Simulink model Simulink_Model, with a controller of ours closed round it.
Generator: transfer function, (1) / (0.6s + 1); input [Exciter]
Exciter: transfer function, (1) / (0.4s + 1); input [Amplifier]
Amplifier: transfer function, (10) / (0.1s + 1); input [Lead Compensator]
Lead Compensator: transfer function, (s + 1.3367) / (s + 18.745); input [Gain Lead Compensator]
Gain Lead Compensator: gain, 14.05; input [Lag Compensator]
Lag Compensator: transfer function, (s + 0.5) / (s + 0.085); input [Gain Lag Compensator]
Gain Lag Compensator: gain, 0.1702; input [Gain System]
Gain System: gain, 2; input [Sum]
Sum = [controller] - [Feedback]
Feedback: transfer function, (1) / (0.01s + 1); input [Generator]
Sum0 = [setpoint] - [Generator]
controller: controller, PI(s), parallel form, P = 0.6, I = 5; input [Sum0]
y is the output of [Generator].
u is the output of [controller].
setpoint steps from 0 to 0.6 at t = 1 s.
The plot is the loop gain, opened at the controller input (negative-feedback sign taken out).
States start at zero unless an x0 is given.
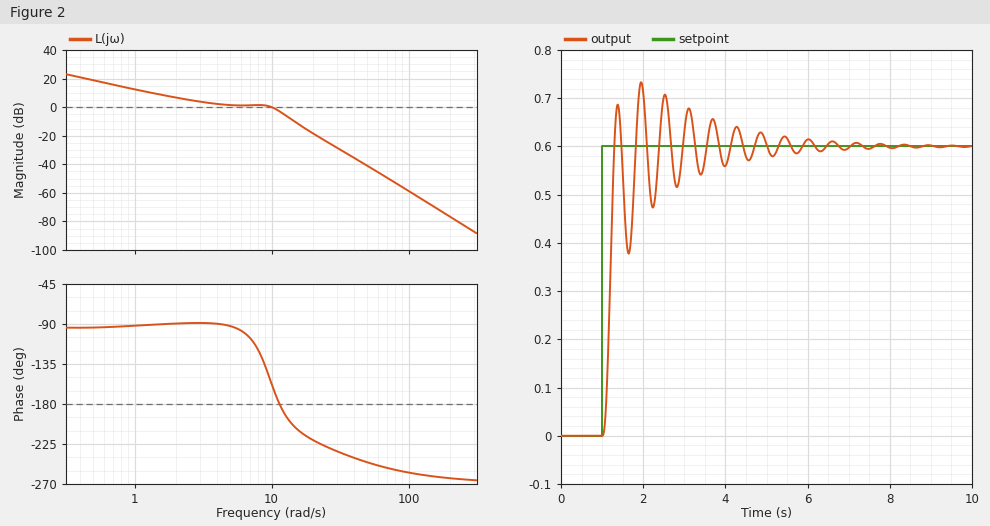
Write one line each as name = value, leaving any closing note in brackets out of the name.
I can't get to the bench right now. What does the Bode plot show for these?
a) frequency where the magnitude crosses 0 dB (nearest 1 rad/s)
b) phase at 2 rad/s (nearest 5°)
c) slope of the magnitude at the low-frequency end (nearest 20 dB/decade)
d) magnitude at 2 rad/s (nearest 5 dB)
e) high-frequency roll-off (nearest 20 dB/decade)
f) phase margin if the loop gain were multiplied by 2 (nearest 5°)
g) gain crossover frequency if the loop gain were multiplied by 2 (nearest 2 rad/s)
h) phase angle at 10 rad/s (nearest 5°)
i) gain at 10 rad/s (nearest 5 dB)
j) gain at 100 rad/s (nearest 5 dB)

frequency where the magnitude crosses 0 dB = 10 rad/s
phase at 2 rad/s = -90°
slope of the magnitude at the low-frequency end = -20 dB/decade
magnitude at 2 rad/s = 5 dB
high-frequency roll-off = -60 dB/decade
phase margin if the loop gain were multiplied by 2 = -15°
gain crossover frequency if the loop gain were multiplied by 2 = 12 rad/s
phase angle at 10 rad/s = -155°
gain at 10 rad/s = 0 dB
gain at 100 rad/s = -60 dB
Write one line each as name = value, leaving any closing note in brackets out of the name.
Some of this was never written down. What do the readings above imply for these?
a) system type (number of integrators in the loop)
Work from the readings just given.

system type = 1
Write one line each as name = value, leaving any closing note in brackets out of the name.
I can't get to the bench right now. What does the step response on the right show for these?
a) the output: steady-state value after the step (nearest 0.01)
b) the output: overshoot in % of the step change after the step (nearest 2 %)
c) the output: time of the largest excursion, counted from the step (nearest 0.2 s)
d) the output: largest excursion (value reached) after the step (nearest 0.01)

the output: steady-state value after the step = 0.60
the output: overshoot in % of the step change after the step = 22 %
the output: time of the largest excursion, counted from the step = 1.0 s
the output: largest excursion (value reached) after the step = 0.73
